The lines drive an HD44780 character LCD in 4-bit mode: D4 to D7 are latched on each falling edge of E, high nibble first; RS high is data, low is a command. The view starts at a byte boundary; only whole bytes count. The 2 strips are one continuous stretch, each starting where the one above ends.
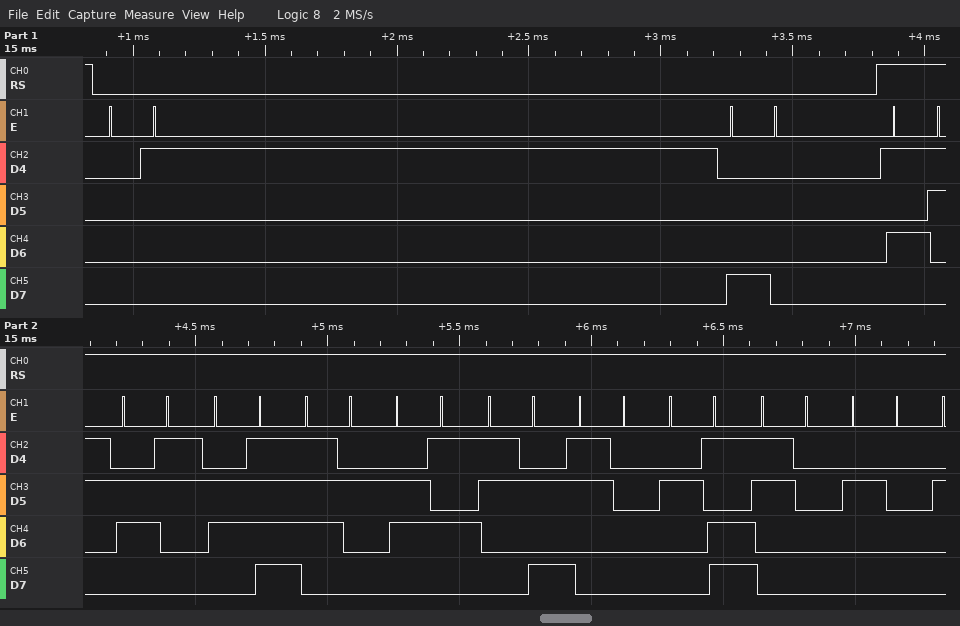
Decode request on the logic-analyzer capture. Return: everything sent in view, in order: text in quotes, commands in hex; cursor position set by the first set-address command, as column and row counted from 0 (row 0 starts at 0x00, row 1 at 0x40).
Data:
0x01 0x80 "Score:0-0 "
column 0, row 0
